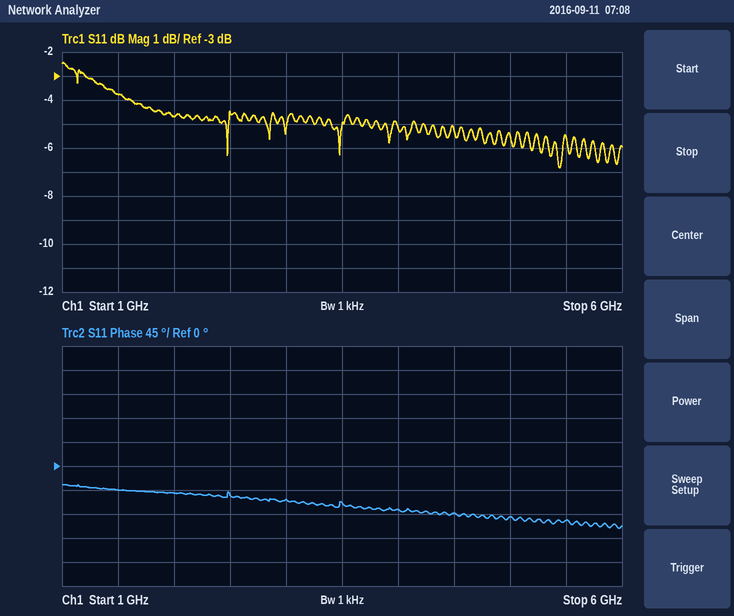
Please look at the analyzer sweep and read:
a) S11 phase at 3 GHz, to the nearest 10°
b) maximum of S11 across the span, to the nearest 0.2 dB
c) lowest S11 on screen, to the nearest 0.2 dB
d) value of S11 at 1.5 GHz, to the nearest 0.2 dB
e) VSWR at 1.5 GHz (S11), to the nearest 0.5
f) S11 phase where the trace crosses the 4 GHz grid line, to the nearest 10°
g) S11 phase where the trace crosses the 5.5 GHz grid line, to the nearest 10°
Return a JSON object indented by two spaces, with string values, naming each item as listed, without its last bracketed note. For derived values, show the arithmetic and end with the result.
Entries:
{
  "S11 phase at 3 GHz, to the nearest 10°": "-60°",
  "maximum of S11 across the span, to the nearest 0.2 dB": "-2.4 dB",
  "lowest S11 on screen, to the nearest 0.2 dB": "-6.8 dB",
  "value of S11 at 1.5 GHz, to the nearest 0.2 dB": "-3.8 dB",
  "VSWR at 1.5 GHz (S11), to the nearest 0.5": "|Γ| = 10^(-3.8/20) = 0.6457; VSWR = (1 + 0.6457)/(1 − 0.6457) ≈ 4.64, so 4.5 to the nearest 0.5",
  "S11 phase where the trace crosses the 4 GHz grid line, to the nearest 10°": "-80°",
  "S11 phase where the trace crosses the 5.5 GHz grid line, to the nearest 10°": "-100°"
}
